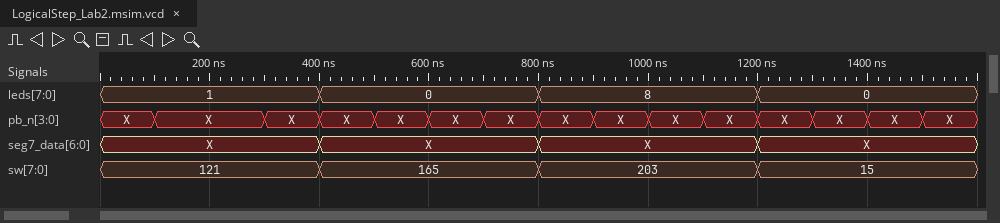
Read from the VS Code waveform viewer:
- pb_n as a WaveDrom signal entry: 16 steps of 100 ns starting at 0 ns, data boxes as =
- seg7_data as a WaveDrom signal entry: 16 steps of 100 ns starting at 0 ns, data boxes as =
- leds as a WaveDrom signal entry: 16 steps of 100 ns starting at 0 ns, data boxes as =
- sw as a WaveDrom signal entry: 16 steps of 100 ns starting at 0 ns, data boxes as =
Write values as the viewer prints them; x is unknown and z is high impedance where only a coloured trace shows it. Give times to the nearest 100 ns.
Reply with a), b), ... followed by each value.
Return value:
a) {name: 'pb_n', wave: '==.=============', data: 'X X X X X X X X X X X X X X X'}
b) {name: 'seg7_data', wave: '=...=...=...=...', data: 'X X X X'}
c) {name: 'leds', wave: '=...=...=...=...', data: '1 0 8 0'}
d) {name: 'sw', wave: '=...=...=...=...', data: '121 165 203 15'}
